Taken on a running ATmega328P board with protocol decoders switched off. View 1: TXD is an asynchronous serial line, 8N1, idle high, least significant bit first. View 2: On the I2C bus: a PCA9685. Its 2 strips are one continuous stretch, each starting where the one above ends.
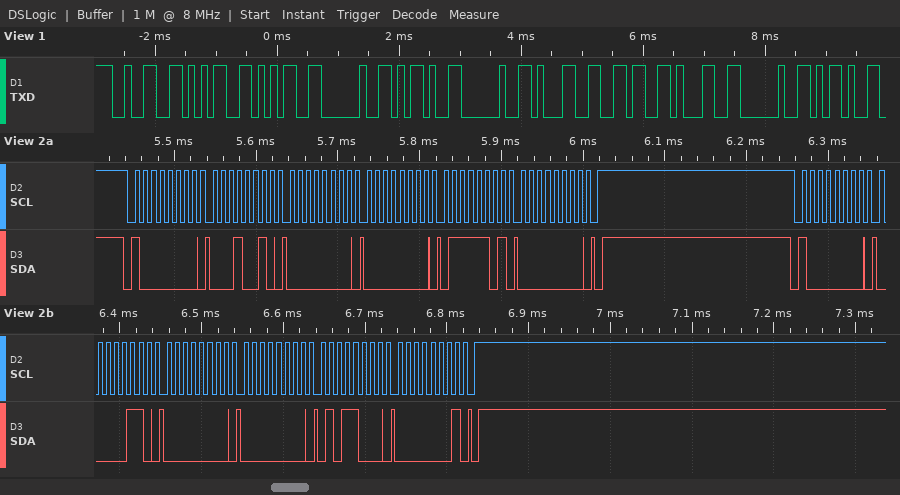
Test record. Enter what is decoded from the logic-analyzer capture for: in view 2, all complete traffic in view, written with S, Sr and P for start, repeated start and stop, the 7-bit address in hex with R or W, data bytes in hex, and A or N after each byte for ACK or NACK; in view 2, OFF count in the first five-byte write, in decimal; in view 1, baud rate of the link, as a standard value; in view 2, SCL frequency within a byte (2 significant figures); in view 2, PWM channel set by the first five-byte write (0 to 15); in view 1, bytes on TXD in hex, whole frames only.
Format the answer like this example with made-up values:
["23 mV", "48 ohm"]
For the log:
["S 40W A 12 A 00 A 00 A 7D A 00 A P S 40W A 06 A 00 A 00 A 58 A 01 A P", "125", "9600 baud", "100 kHz", "3", "0x32 0x35 0x35 0x20 0x2D 0x20 0x31 0x36 0x31 0x20 0x2D"]
